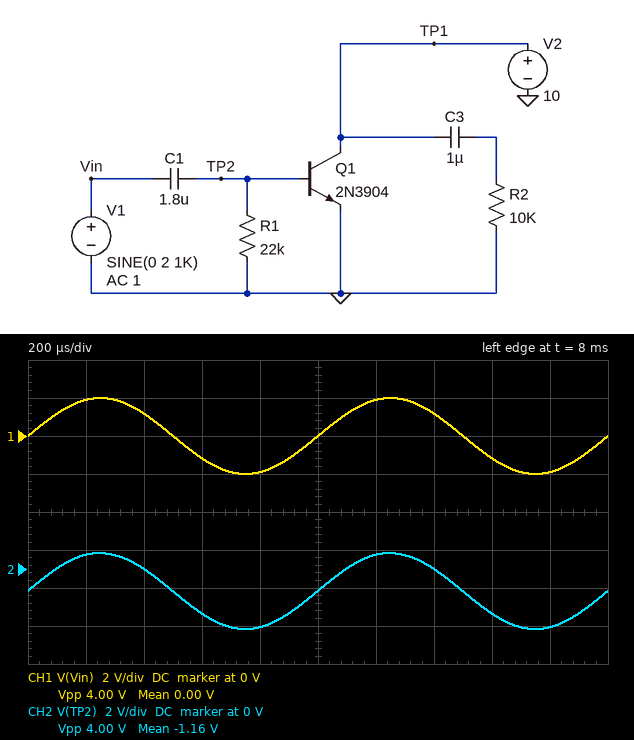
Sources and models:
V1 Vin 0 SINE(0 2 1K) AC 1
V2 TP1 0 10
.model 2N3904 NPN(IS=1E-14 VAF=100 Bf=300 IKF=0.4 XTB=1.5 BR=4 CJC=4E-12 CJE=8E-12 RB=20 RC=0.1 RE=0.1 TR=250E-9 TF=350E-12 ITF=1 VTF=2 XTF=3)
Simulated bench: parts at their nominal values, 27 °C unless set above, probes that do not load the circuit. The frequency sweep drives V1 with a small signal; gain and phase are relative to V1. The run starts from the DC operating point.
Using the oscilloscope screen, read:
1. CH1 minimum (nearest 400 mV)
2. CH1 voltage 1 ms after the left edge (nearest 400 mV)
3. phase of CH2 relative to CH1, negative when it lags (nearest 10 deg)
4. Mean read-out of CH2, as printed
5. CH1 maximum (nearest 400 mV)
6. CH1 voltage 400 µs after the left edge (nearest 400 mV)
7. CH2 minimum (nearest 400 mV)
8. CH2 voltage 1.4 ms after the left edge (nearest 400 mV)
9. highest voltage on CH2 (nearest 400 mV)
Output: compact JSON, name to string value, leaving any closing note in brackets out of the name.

{"CH1 minimum": "-2.0 V", "CH1 voltage 1 ms after the left edge": "0 V", "phase of CH2 relative to CH1, negative when it lags": "0 deg", "Mean read-out of CH2, as printed": "-1.16 V", "CH1 maximum": "2.0 V", "CH1 voltage 400 µs after the left edge": "1.2 V", "CH2 minimum": "-3.2 V", "CH2 voltage 1.4 ms after the left edge": "0 V", "highest voltage on CH2": "800 mV"}
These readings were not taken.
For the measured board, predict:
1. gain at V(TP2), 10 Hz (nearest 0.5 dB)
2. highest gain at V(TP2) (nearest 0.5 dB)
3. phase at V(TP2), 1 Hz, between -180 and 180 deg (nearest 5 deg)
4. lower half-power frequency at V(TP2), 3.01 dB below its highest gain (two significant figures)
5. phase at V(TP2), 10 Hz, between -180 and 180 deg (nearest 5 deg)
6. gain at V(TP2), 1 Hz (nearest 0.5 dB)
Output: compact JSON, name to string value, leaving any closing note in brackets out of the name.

{"gain at V(TP2), 10 Hz": "-0.5 dB", "highest gain at V(TP2)": "0 dB", "phase at V(TP2), 1 Hz, between -180 and 180 deg": "75 deg", "lower half-power frequency at V(TP2), 3.01 dB below its highest gain": "4.0 Hz", "phase at V(TP2), 10 Hz, between -180 and 180 deg": "20 deg", "gain at V(TP2), 1 Hz": "-12.5 dB"}
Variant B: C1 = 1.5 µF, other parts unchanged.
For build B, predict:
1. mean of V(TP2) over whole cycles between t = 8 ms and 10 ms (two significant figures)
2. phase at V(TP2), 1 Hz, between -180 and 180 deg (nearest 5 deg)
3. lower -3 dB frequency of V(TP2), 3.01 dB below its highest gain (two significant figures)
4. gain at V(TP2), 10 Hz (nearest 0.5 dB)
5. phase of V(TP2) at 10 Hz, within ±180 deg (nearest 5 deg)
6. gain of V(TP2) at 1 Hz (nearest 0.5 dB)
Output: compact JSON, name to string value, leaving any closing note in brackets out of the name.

{"mean of V(TP2) over whole cycles between t = 8 ms and 10 ms": "-1.2 V", "phase at V(TP2), 1 Hz, between -180 and 180 deg": "80 deg", "lower -3 dB frequency of V(TP2), 3.01 dB below its highest gain": "4.8 Hz", "gain at V(TP2), 10 Hz": "-1.0 dB", "phase of V(TP2) at 10 Hz, within ±180 deg": "25 deg", "gain of V(TP2) at 1 Hz": "-14.0 dB"}
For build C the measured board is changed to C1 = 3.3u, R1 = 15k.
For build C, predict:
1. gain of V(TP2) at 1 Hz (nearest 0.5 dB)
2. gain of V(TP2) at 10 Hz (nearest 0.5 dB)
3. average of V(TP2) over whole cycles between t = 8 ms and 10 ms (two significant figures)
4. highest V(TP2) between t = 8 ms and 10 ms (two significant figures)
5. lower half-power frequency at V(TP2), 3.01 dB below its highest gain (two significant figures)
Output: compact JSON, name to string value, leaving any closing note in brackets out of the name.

{"gain of V(TP2) at 1 Hz": "-10.5 dB", "gain of V(TP2) at 10 Hz": "-0.5 dB", "average of V(TP2) over whole cycles between t = 8 ms and 10 ms": "-1.1 V", "highest V(TP2) between t = 8 ms and 10 ms": "860 mV", "lower half-power frequency at V(TP2), 3.01 dB below its highest gain": "3.2 Hz"}
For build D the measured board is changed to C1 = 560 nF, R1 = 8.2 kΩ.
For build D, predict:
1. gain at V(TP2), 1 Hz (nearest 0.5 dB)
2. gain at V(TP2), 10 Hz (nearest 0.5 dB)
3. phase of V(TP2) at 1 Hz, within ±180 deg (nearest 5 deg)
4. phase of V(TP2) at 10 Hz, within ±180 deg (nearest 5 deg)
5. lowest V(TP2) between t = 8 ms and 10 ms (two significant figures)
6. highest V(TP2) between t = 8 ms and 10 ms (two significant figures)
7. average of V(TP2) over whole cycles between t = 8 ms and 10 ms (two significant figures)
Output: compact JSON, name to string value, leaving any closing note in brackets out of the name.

{"gain at V(TP2), 1 Hz": "-31.0 dB", "gain at V(TP2), 10 Hz": "-11.0 dB", "phase of V(TP2) at 1 Hz, within ±180 deg": "90 deg", "phase of V(TP2) at 10 Hz, within ±180 deg": "75 deg", "lowest V(TP2) between t = 8 ms and 10 ms": "-3.1 V", "highest V(TP2) between t = 8 ms and 10 ms": "890 mV", "average of V(TP2) over whole cycles between t = 8 ms and 10 ms": "-1.1 V"}
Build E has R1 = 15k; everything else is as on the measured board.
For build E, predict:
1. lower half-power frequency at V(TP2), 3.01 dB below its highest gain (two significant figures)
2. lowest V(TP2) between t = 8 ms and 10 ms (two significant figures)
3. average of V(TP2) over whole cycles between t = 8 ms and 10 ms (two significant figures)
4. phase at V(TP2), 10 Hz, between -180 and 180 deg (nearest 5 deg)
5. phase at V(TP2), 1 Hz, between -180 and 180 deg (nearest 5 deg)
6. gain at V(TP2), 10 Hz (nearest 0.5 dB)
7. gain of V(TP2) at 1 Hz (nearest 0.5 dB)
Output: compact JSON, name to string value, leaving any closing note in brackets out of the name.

{"lower half-power frequency at V(TP2), 3.01 dB below its highest gain": "5.9 Hz", "lowest V(TP2) between t = 8 ms and 10 ms": "-3.1 V", "average of V(TP2) over whole cycles between t = 8 ms and 10 ms": "-1.1 V", "phase at V(TP2), 10 Hz, between -180 and 180 deg": "30 deg", "phase at V(TP2), 1 Hz, between -180 and 180 deg": "80 deg", "gain at V(TP2), 10 Hz": "-1.5 dB", "gain of V(TP2) at 1 Hz": "-15.5 dB"}
